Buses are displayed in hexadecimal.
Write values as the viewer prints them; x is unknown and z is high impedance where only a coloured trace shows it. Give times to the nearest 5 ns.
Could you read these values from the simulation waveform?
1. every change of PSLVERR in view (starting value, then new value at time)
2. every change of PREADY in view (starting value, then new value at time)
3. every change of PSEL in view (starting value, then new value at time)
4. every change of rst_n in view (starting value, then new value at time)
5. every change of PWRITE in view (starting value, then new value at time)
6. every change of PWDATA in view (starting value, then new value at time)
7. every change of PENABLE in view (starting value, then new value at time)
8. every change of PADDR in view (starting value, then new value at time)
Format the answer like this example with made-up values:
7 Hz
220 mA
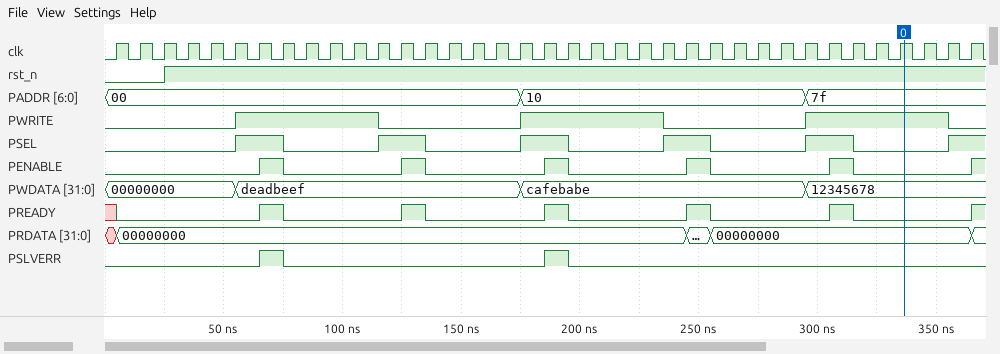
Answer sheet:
0, 1 at 65 ns, 0 at 75 ns, 1 at 185 ns, 0 at 195 ns
x, 0 at 5 ns, 1 at 65 ns, 0 at 75 ns, 1 at 125 ns, 0 at 135 ns, 1 at 185 ns, 0 at 195 ns, 1 at 245 ns, 0 at 255 ns, 1 at 305 ns, 0 at 315 ns, 1 at 365 ns
0, 1 at 55 ns, 0 at 75 ns, 1 at 115 ns, 0 at 135 ns, 1 at 175 ns, 0 at 195 ns, 1 at 235 ns, 0 at 255 ns, 1 at 295 ns, 0 at 315 ns, 1 at 355 ns
0, 1 at 25 ns
0, 1 at 55 ns, 0 at 115 ns, 1 at 175 ns, 0 at 235 ns, 1 at 295 ns, 0 at 355 ns
00000000, deadbeef at 55 ns, cafebabe at 175 ns, 12345678 at 295 ns
0, 1 at 65 ns, 0 at 75 ns, 1 at 125 ns, 0 at 135 ns, 1 at 185 ns, 0 at 195 ns, 1 at 245 ns, 0 at 255 ns, 1 at 305 ns, 0 at 315 ns, 1 at 365 ns
00, 10 at 175 ns, 7f at 295 ns
